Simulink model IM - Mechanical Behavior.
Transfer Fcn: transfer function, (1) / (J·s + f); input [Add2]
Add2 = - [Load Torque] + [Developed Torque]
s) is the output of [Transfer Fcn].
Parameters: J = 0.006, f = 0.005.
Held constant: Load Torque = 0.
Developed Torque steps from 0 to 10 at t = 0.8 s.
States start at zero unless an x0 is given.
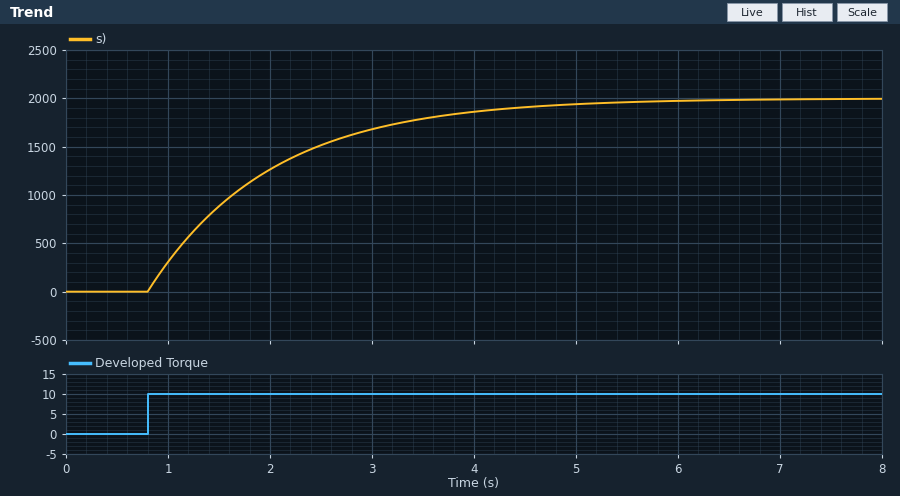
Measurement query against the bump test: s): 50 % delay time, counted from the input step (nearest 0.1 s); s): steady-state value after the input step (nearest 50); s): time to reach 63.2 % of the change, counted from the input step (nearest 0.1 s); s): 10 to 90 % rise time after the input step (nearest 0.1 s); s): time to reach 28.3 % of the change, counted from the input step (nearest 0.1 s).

0.8 s
2000
1.2 s
2.6 s
0.4 s
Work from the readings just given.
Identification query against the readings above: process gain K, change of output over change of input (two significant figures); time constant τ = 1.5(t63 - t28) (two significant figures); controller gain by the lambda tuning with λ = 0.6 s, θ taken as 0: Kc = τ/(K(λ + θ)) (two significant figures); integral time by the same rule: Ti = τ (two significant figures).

200
1.2 s
0.010
1.2 s
